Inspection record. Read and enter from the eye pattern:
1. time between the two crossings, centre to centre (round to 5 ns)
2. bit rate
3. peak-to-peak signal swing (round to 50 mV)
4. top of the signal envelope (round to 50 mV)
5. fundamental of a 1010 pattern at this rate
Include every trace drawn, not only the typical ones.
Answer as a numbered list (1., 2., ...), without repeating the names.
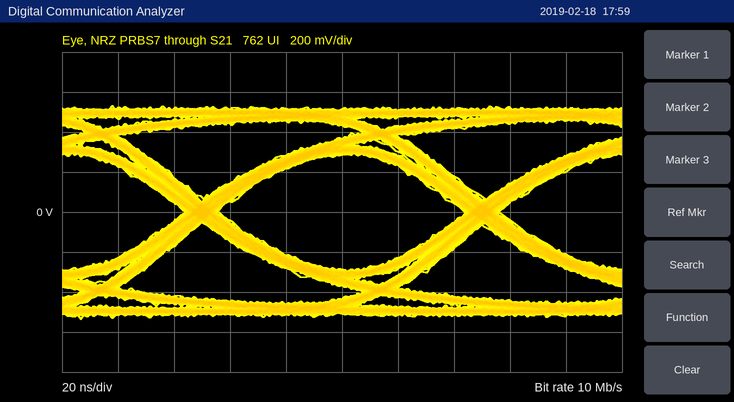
1. 100 ns
2. 10 Mb/s
3. 1.05 V
4. 550 mV
5. 5 MHz
